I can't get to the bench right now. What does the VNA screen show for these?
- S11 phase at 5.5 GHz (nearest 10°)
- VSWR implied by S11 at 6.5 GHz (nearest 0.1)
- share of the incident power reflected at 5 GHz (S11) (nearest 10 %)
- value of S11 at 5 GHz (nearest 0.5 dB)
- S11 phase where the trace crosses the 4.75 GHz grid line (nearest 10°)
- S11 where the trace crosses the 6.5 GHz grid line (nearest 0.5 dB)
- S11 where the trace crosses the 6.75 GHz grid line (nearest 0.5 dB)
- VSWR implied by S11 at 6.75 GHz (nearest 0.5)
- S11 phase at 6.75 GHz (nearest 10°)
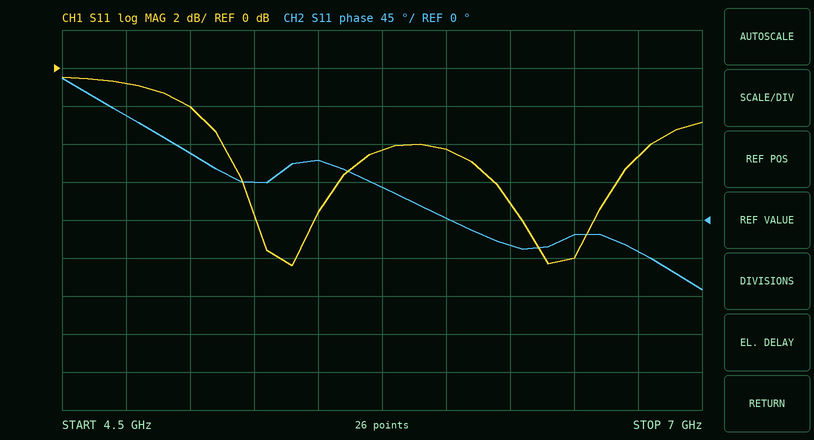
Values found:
70°
1.9
60 %
-2.0 dB
120°
-10.0 dB
-4.5 dB
4.0
-40°
